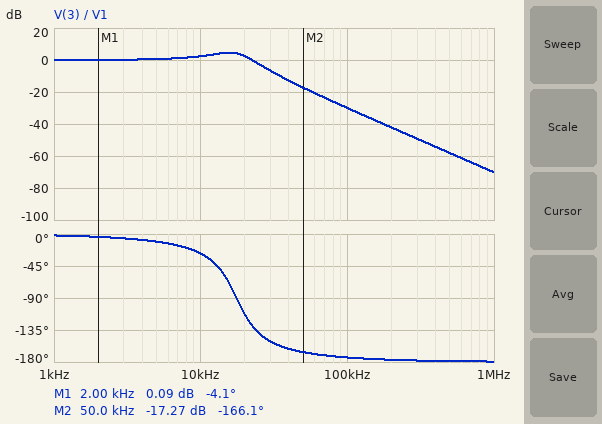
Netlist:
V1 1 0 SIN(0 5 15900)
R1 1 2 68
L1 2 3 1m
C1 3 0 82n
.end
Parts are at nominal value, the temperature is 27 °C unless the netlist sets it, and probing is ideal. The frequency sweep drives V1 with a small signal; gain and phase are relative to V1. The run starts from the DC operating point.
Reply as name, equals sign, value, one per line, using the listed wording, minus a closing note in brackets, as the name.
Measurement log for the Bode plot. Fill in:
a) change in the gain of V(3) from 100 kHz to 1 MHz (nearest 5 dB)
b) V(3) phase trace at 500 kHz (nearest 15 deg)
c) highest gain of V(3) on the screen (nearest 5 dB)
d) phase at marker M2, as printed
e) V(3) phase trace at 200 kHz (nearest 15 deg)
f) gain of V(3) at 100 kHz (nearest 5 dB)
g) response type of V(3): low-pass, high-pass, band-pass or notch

change in the gain of V(3) from 100 kHz to 1 MHz = -40 dB
V(3) phase trace at 500 kHz = -180 deg
highest gain of V(3) on the screen = 5 dB
phase at marker M2, as printed = -166.1 deg
V(3) phase trace at 200 kHz = -180 deg
gain of V(3) at 100 kHz = -30 dB
response type of V(3): low-pass, high-pass, band-pass or notch = low-pass
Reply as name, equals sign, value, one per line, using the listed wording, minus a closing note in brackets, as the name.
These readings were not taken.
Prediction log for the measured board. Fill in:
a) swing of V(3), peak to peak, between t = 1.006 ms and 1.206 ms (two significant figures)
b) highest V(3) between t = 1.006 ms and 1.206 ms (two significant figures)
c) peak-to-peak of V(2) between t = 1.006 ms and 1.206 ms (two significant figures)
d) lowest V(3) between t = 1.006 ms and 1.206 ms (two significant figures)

swing of V(3), peak to peak, between t = 1.006 ms and 1.206 ms = 17 V
highest V(3) between t = 1.006 ms and 1.206 ms = 8.5 V
peak-to-peak of V(2) between t = 1.006 ms and 1.206 ms = 3.1 V
lowest V(3) between t = 1.006 ms and 1.206 ms = -8.5 V
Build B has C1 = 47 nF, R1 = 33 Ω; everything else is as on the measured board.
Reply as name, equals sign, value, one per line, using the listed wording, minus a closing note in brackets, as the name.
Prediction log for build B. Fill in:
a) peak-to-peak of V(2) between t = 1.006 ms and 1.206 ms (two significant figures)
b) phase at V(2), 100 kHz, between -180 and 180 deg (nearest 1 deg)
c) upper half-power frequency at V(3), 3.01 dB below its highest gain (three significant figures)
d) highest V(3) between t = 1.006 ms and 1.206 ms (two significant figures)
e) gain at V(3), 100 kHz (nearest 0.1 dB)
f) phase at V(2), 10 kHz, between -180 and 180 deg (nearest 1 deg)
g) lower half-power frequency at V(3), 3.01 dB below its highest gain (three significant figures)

peak-to-peak of V(2) between t = 1.006 ms and 1.206 ms = 9.6 V
phase at V(2), 100 kHz, between -180 and 180 deg = 3 deg
upper half-power frequency at V(3), 3.01 dB below its highest gain = 25.4 kHz
highest V(3) between t = 1.006 ms and 1.206 ms = 9.0 V
gain at V(3), 100 kHz = -24.9 dB
phase at V(2), 10 kHz, between -180 and 180 deg = -7 deg
lower half-power frequency at V(3), 3.01 dB below its highest gain = 20.1 kHz
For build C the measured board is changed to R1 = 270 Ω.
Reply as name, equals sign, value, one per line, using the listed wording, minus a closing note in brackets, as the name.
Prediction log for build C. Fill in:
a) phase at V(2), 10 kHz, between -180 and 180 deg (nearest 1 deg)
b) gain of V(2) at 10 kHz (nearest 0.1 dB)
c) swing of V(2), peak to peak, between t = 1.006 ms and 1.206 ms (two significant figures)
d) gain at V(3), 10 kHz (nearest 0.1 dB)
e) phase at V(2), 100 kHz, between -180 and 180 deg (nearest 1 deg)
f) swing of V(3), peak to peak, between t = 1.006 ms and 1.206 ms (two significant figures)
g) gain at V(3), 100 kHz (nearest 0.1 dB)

phase at V(2), 10 kHz, between -180 and 180 deg = -64 deg
gain of V(2) at 10 kHz = -7.2 dB
swing of V(2), peak to peak, between t = 1.006 ms and 1.206 ms = 820 mV
gain at V(3), 10 kHz = -3.8 dB
phase at V(2), 100 kHz, between -180 and 180 deg = 24 deg
swing of V(3), peak to peak, between t = 1.006 ms and 1.206 ms = 4.5 V
gain at V(3), 100 kHz = -30.7 dB
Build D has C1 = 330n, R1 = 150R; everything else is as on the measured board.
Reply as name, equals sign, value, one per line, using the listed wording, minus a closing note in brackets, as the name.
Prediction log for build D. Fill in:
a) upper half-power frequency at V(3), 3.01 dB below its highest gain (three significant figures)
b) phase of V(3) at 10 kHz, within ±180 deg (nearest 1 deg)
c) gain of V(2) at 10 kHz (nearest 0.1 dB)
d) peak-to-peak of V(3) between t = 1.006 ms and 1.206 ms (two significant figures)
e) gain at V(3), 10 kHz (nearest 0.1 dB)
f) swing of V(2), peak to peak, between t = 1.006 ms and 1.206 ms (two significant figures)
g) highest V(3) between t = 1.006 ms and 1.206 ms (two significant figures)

upper half-power frequency at V(3), 3.01 dB below its highest gain = 3.70 kHz
phase of V(3) at 10 kHz, within ±180 deg = -96 deg
gain of V(2) at 10 kHz = -20.3 dB
peak-to-peak of V(3) between t = 1.006 ms and 1.206 ms = 1.8 V
gain at V(3), 10 kHz = -9.9 dB
swing of V(2), peak to peak, between t = 1.006 ms and 1.206 ms = 4.2 V
highest V(3) between t = 1.006 ms and 1.206 ms = 920 mV
